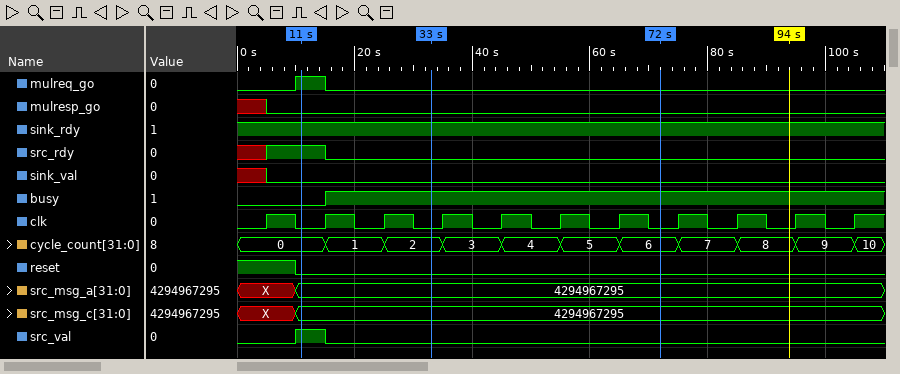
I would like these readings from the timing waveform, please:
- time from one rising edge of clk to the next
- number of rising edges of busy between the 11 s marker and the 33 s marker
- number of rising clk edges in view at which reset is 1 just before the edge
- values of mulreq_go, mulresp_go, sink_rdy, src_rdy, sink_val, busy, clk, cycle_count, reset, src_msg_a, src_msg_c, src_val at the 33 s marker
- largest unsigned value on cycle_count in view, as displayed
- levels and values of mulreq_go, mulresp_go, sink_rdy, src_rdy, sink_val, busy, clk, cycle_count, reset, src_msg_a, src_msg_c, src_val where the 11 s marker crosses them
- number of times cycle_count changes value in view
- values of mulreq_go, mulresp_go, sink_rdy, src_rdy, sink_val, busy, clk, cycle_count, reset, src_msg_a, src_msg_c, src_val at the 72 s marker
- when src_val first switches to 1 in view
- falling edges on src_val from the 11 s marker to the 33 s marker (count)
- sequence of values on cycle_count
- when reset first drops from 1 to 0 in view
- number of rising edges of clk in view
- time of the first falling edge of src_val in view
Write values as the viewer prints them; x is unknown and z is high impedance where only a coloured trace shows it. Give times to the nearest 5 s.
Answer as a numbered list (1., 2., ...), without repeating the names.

1. 10 s
2. 1
3. 1
4. mulreq_go=0, mulresp_go=0, sink_rdy=1, src_rdy=0, sink_val=0, busy=1, clk=0, cycle_count=2, reset=0, src_msg_a=4294967295, src_msg_c=4294967295, src_val=0
5. 10
6. mulreq_go=1, mulresp_go=0, sink_rdy=1, src_rdy=1, sink_val=0, busy=0, clk=0, cycle_count=0, reset=0, src_msg_a=4294967295, src_msg_c=4294967295, src_val=1
7. 10
8. mulreq_go=0, mulresp_go=0, sink_rdy=1, src_rdy=0, sink_val=0, busy=1, clk=0, cycle_count=6, reset=0, src_msg_a=4294967295, src_msg_c=4294967295, src_val=0
9. 10 s
10. 1
11. 0, 1, 2, 3, 4, 5, 6, 7, 8, 9, 10
12. 10 s
13. 11
14. 15 s
